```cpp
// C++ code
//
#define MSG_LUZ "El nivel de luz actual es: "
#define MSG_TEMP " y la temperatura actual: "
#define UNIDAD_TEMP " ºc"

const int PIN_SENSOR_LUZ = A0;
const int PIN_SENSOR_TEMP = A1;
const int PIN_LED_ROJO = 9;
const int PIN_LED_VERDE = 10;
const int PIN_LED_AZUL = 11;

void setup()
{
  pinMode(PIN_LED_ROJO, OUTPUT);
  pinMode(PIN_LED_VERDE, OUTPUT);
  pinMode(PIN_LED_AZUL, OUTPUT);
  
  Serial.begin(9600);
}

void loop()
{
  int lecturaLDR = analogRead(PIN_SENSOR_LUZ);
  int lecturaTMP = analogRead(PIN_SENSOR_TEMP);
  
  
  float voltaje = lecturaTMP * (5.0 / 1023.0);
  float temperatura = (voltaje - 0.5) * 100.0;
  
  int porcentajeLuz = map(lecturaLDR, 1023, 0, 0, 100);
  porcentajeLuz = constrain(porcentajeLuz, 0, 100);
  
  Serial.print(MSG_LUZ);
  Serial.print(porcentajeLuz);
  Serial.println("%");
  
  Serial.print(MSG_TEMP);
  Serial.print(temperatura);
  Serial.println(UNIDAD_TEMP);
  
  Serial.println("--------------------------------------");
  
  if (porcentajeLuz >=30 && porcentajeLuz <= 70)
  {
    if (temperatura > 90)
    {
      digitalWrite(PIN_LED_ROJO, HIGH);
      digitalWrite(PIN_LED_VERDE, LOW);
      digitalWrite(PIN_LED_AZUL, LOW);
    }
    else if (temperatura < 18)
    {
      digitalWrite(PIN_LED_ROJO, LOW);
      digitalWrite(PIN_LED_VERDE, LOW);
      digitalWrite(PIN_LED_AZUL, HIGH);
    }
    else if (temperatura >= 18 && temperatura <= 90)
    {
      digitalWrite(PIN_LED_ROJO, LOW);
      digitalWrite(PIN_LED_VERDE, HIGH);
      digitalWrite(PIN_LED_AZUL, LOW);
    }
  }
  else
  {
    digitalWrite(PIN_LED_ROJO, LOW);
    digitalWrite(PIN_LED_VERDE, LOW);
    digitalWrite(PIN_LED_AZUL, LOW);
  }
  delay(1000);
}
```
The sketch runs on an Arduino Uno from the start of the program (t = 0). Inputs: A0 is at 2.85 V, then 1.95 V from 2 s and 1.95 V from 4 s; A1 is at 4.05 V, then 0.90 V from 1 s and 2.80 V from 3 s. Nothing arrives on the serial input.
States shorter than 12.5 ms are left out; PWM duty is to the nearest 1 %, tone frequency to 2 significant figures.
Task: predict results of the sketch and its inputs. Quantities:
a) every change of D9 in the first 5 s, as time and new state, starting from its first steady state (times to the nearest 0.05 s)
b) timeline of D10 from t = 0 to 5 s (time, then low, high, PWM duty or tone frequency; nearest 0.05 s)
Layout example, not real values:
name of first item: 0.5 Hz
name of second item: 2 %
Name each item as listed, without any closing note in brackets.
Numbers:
every change of D9 in the first 5 s, as time and new state, starting from its first steady state: 0 s low; 0.05 s high; 1.1 s low; 3.2 s high
timeline of D10 from t = 0 to 5 s: 0 s low; 1.1 s high; 3.2 s low
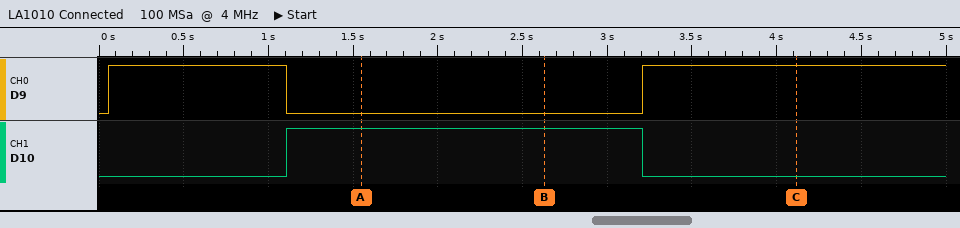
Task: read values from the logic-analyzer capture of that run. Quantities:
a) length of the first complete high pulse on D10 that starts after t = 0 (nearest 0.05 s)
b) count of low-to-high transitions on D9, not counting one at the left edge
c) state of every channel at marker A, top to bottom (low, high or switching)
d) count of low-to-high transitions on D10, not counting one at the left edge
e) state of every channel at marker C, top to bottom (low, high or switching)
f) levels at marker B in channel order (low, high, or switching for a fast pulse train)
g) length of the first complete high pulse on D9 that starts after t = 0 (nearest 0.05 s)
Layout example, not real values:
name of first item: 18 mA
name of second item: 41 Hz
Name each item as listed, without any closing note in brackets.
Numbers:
length of the first complete high pulse on D10 that starts after t = 0: 2.10 s
count of low-to-high transitions on D9, not counting one at the left edge: 2
state of every channel at marker A, top to bottom: D9 low, D10 high
count of low-to-high transitions on D10, not counting one at the left edge: 1
state of every channel at marker C, top to bottom: D9 high, D10 low
levels at marker B in channel order: D9 low, D10 high
length of the first complete high pulse on D9 that starts after t = 0: 1.05 s
